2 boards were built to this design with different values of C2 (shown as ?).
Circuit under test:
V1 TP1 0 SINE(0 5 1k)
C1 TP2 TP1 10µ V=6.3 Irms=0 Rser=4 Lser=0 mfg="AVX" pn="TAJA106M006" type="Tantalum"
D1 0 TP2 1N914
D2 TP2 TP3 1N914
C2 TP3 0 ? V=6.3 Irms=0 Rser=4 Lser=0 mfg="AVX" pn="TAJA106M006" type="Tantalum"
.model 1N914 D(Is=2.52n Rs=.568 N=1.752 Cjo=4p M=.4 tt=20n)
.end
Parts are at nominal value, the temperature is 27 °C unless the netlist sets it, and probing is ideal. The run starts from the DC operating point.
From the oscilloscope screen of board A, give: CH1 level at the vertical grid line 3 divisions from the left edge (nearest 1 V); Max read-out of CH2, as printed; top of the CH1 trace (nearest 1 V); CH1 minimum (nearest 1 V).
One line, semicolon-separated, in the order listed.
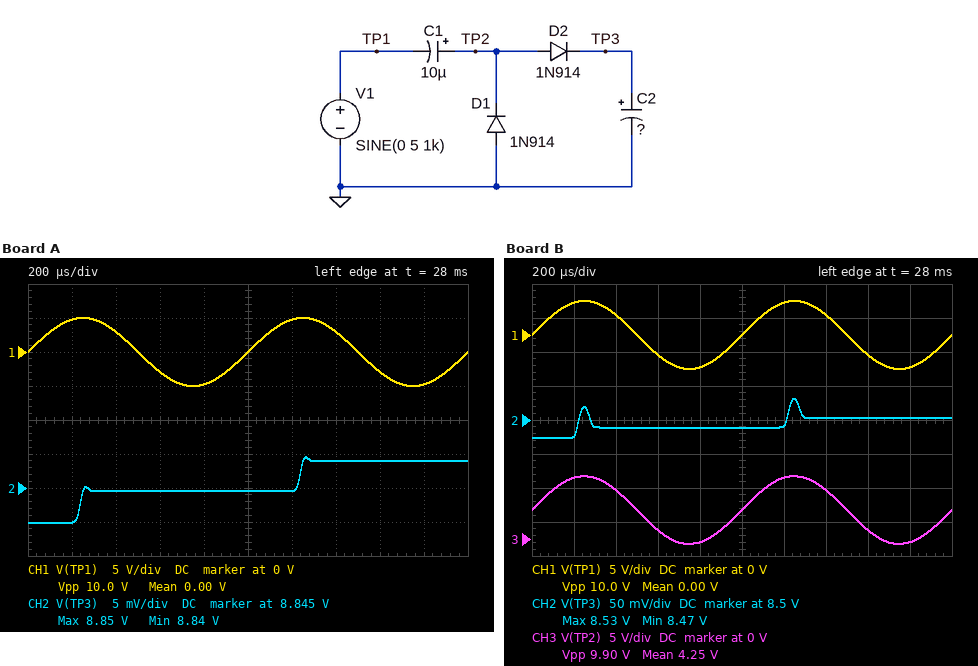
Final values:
-3 V; 8.85 V; 5 V; -5 V
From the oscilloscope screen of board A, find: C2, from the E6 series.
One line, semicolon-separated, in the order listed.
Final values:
4.7 µF
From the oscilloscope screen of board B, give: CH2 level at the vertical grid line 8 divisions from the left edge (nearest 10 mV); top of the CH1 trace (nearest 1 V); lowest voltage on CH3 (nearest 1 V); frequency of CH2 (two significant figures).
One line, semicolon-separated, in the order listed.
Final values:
8.50 V; 5 V; -1 V; 1.0 kHz
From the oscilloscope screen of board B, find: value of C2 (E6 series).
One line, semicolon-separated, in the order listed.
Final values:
33 µF
